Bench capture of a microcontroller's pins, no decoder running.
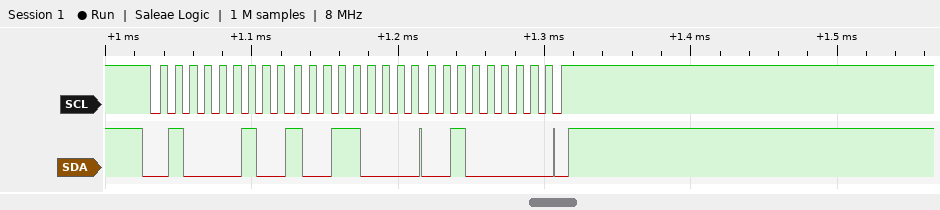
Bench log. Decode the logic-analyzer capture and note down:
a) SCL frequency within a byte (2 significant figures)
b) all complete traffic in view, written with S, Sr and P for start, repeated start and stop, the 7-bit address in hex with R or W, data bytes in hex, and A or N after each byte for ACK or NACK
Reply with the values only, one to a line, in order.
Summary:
100 kHz
S 21W A 98 A 20 A P
